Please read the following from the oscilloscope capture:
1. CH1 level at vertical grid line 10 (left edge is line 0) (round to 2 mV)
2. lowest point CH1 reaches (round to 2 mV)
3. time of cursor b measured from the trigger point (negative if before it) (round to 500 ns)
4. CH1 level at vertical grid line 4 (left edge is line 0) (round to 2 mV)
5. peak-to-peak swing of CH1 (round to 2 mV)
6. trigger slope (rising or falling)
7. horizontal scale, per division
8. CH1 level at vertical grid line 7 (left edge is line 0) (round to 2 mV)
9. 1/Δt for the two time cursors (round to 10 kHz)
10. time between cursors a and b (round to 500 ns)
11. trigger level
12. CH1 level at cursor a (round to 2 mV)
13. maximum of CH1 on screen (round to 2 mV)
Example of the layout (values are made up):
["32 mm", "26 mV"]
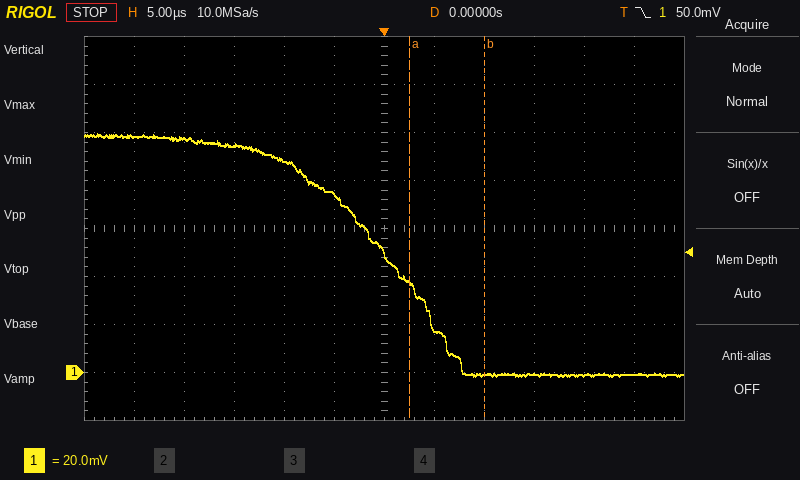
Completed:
["-2 mV", "-2 mV", "+10.0 µs", "88 mV", "102 mV", "falling", "5 µs", "18 mV", "130 kHz", "7.5 µs", "50.0 mV", "38 mV", "100 mV"]
